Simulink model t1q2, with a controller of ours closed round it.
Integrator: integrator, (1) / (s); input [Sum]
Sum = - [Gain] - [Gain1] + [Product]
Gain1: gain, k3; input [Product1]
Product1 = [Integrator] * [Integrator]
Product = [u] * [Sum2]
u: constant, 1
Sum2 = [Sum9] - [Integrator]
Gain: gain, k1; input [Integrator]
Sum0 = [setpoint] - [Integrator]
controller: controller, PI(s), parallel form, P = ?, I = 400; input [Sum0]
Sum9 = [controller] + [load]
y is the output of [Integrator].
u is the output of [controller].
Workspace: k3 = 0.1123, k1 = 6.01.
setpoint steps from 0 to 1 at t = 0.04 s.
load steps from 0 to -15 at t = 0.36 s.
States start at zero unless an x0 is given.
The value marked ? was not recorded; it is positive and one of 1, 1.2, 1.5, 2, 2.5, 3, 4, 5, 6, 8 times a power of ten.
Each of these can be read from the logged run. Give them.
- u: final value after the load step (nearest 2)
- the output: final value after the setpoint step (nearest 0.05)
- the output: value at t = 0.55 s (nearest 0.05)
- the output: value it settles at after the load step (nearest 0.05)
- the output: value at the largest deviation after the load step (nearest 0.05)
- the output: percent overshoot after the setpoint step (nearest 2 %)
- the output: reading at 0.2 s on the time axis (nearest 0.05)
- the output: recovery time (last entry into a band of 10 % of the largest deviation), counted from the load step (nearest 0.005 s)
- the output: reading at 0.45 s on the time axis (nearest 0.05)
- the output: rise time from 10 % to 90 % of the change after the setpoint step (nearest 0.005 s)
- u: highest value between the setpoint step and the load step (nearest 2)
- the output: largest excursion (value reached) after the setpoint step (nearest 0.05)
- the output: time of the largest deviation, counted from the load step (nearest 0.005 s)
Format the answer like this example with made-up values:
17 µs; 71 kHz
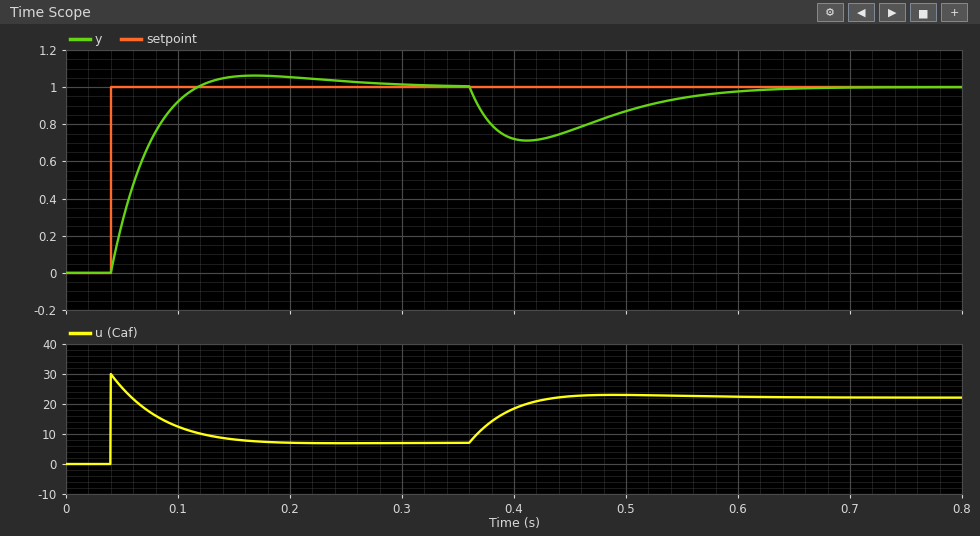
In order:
22; 1.00; 0.95; 1.00; 0.70; 6 %; 1.05; 0.230 s; 0.75; 0.055 s; 30; 1.05; 0.050 s
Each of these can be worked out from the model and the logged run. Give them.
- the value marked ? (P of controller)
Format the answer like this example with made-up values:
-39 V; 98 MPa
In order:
30
